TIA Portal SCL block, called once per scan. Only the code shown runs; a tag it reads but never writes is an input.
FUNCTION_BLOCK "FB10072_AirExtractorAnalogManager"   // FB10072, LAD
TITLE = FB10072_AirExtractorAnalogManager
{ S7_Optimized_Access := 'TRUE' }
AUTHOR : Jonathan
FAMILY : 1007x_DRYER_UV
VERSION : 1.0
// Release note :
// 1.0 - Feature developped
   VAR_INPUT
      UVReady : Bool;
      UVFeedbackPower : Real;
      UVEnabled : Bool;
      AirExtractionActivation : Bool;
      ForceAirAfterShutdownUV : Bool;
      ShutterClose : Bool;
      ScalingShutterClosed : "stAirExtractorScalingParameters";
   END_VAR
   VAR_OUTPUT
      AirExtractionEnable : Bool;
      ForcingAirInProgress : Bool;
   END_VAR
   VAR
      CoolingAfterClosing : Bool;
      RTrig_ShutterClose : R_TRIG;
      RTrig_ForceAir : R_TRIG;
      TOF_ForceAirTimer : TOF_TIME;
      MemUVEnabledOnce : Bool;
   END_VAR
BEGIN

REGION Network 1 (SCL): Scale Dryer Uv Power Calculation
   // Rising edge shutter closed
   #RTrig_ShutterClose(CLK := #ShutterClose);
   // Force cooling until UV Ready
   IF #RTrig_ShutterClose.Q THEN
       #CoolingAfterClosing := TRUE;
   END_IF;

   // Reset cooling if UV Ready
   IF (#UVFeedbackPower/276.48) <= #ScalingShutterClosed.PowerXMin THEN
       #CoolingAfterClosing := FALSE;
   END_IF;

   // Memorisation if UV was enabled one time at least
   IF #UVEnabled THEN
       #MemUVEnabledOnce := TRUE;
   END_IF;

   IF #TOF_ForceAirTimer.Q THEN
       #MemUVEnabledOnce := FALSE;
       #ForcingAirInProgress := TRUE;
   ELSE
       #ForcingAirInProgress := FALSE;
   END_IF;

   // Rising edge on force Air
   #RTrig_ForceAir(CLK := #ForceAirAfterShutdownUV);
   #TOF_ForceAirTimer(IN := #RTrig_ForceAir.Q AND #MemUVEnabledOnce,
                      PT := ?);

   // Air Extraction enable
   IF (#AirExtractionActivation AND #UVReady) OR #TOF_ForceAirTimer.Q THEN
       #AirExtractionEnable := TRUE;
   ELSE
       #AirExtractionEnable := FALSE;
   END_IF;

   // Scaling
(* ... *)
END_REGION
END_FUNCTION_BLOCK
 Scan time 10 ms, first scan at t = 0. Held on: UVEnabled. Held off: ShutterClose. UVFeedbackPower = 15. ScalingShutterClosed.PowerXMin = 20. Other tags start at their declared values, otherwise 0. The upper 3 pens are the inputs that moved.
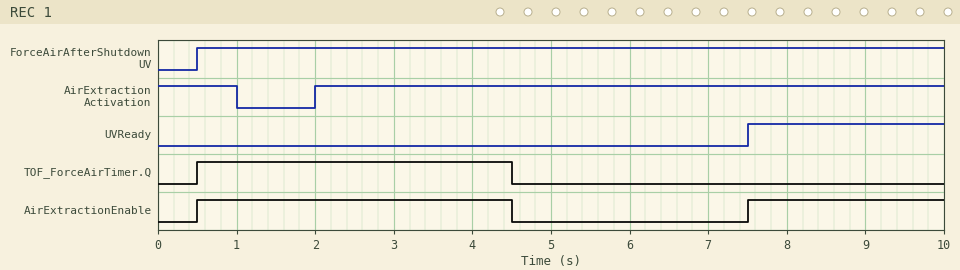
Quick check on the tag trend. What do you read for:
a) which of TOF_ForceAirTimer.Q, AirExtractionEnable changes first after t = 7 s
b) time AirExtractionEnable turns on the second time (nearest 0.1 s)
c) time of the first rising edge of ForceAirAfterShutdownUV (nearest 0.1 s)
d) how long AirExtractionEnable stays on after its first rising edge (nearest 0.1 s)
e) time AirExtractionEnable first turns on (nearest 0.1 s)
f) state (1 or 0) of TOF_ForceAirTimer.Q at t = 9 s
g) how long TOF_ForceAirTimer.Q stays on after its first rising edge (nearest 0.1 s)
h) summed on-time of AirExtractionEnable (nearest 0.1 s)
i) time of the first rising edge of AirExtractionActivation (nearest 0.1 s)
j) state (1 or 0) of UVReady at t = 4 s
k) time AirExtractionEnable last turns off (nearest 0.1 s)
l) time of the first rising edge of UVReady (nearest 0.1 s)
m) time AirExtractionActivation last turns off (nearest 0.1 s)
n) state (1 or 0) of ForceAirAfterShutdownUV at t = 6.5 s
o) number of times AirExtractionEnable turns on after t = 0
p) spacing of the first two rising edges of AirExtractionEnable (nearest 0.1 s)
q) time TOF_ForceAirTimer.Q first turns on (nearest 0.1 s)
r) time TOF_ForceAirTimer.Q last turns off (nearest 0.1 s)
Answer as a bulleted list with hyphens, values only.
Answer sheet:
- AirExtractionEnable
- 7.5 s
- 0.5 s
- 4.0 s
- 0.5 s
- 0
- 4.0 s
- 6.5 s
- 2.0 s
- 0
- 4.5 s
- 7.5 s
- 1.0 s
- 1
- 2
- 7.0 s
- 0.5 s
- 4.5 s
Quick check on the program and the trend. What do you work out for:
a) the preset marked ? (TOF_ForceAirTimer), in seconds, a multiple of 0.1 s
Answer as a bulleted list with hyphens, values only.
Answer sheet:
- 4.0 s
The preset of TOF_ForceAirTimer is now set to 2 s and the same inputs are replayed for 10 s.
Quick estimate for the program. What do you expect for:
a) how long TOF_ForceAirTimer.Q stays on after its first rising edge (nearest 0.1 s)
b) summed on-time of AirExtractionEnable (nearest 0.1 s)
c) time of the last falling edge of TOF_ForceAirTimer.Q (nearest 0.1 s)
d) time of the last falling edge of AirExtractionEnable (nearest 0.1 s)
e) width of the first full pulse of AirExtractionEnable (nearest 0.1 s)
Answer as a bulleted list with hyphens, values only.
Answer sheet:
- 2.0 s
- 4.5 s
- 2.5 s
- 2.5 s
- 2.0 s
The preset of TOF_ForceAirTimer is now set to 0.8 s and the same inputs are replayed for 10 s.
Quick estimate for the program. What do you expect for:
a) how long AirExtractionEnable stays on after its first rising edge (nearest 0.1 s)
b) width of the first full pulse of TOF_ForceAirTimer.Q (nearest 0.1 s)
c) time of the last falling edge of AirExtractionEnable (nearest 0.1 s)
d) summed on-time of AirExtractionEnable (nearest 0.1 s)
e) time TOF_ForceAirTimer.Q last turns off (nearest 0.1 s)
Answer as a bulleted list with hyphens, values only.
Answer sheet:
- 0.8 s
- 0.8 s
- 1.3 s
- 3.3 s
- 1.3 s
